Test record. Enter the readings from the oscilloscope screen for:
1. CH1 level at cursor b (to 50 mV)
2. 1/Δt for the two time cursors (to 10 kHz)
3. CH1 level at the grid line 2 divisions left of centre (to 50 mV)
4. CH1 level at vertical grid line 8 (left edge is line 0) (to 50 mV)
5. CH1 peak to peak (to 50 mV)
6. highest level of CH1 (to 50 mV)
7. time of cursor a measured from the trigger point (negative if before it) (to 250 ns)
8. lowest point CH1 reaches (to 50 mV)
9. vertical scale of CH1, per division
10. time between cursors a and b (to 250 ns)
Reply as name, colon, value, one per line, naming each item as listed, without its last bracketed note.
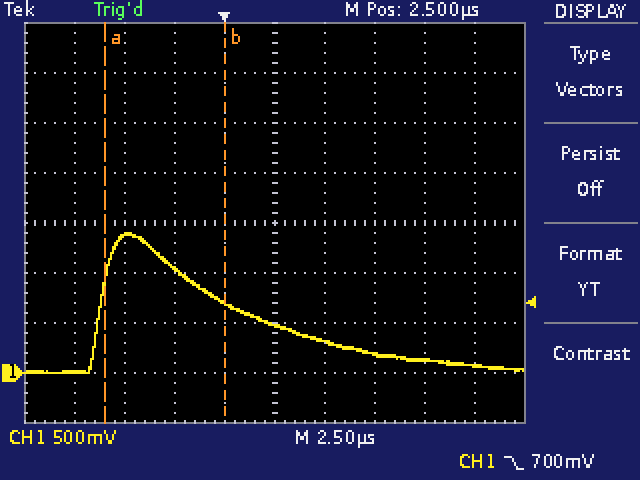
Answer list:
CH1 level at cursor b: 700 mV
1/Δt for the two time cursors: 170 kHz
CH1 level at the grid line 2 divisions left of centre: 1.05 V
CH1 level at vertical grid line 8 (left edge is line 0): 150 mV
CH1 peak to peak: 1.40 V
highest level of CH1: 1.40 V
time of cursor a measured from the trigger point (negative if before it): -6.00 µs
lowest point CH1 reaches: 0 mV
vertical scale of CH1, per division: 500 mV
time between cursors a and b: 6.00 µs
